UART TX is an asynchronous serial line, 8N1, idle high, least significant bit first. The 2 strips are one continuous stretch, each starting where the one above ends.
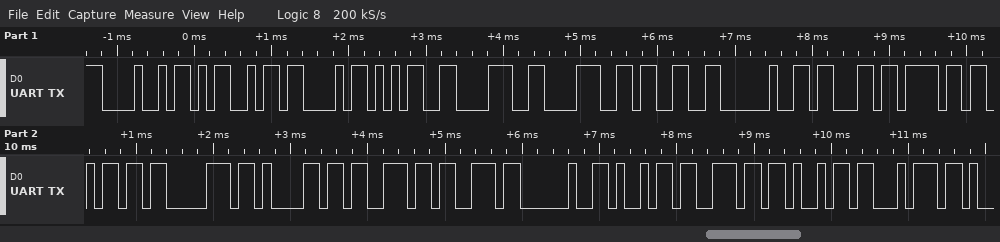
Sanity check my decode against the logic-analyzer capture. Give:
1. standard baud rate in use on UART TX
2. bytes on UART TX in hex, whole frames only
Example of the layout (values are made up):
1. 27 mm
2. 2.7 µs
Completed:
1. 9600 baud
2. 0x48 0x4D 0x43 0x35 0x38 0x38 0x33 0x20 0x63 0x6F 0x6D 0x70 0x61 0x73 0x73 0x20 0x69 0x6E 0x69 0x74
